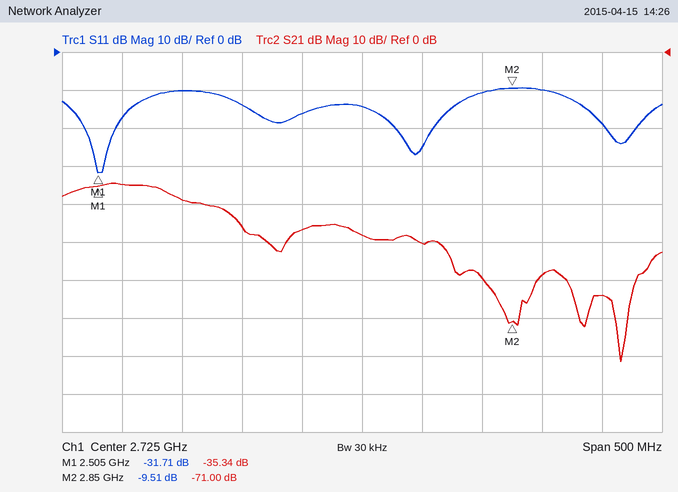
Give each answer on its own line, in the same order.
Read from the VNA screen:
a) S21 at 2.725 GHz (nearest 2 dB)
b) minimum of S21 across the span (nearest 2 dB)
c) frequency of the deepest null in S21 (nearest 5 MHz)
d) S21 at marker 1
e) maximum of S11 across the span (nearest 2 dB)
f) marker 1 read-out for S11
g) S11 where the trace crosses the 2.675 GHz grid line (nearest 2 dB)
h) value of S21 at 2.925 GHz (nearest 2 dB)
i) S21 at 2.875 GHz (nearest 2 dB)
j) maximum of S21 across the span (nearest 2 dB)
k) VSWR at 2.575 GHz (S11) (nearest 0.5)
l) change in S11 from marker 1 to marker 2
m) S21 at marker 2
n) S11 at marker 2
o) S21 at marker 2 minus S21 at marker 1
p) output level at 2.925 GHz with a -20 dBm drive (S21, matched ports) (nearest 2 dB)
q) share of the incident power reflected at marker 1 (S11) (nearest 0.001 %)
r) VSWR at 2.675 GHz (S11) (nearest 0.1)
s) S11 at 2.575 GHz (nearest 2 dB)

-48 dB
-82 dB
2.940 GHz
-35.34 dB
-10 dB
-31.71 dB
-16 dB
-64 dB
-58 dB
-34 dB
2.0
22.20 dB
-71.00 dB
-9.51 dB
-35.66 dB
-84 dBm
0.067 %
1.4
-10 dB
